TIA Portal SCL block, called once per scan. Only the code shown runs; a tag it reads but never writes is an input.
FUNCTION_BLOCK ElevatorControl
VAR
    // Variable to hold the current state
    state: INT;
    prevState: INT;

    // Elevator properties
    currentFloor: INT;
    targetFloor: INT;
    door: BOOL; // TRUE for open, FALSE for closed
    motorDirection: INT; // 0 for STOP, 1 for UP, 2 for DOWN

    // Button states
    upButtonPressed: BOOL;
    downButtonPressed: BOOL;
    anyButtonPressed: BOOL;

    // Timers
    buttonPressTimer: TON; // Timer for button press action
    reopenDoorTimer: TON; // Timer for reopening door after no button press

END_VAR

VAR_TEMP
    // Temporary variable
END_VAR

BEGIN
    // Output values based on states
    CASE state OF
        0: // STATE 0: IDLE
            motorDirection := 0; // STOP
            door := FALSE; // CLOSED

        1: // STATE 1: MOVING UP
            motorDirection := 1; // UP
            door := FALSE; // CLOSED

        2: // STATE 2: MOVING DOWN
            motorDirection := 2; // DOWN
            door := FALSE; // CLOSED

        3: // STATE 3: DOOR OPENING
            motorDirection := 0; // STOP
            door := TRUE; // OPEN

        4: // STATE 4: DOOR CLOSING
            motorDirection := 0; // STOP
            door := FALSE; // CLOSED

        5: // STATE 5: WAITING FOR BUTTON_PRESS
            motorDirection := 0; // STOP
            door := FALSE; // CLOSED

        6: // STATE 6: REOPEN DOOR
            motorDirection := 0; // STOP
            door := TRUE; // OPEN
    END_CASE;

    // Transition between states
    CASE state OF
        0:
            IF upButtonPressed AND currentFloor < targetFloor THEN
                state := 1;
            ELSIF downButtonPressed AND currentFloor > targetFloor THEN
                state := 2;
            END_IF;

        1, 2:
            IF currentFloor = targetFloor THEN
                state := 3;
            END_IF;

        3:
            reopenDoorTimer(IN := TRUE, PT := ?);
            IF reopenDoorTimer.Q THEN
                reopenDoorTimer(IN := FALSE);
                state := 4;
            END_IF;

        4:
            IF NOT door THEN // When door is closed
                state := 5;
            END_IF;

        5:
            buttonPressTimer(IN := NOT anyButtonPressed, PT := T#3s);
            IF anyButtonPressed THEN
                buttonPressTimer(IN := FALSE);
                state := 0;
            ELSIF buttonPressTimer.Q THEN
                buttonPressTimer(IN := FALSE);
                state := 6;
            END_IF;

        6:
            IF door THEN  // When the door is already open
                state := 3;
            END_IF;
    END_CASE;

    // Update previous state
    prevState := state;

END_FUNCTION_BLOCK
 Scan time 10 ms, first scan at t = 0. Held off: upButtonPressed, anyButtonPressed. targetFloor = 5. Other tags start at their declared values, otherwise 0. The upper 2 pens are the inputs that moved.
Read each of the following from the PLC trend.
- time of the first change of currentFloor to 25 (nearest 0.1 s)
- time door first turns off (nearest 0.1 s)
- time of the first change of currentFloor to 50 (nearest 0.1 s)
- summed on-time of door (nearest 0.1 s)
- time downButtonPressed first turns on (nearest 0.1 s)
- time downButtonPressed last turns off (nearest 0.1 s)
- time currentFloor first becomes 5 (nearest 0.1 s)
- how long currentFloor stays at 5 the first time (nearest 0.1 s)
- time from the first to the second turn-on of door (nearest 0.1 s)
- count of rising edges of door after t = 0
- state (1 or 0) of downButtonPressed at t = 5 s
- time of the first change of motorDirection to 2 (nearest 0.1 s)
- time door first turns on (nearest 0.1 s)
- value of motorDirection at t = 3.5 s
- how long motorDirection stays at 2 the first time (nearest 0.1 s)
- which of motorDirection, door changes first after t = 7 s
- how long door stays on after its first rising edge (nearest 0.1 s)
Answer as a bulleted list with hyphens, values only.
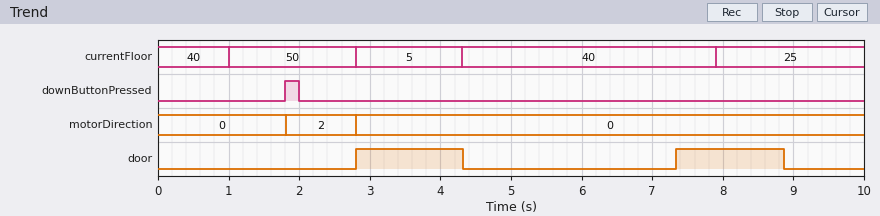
- 7.9 s
- 4.3 s
- 1.0 s
- 3.0 s
- 1.8 s
- 2.0 s
- 2.8 s
- 1.5 s
- 4.5 s
- 2
- 0
- 1.8 s
- 2.8 s
- 0
- 1.0 s
- door
- 1.5 s
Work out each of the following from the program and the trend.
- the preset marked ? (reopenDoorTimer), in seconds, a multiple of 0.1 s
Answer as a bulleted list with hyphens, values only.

- 1.5 s
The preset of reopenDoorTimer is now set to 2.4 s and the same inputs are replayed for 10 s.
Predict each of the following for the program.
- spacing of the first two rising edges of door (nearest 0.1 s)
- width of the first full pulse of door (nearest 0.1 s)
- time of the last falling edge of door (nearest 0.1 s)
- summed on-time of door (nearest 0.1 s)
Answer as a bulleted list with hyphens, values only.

- 5.4 s
- 2.4 s
- 5.2 s
- 4.2 s
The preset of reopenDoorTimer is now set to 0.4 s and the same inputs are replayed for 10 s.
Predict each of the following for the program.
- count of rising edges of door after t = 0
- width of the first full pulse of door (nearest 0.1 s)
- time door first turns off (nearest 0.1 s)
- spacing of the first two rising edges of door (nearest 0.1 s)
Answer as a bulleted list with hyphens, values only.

- 3
- 0.4 s
- 3.2 s
- 3.4 s
